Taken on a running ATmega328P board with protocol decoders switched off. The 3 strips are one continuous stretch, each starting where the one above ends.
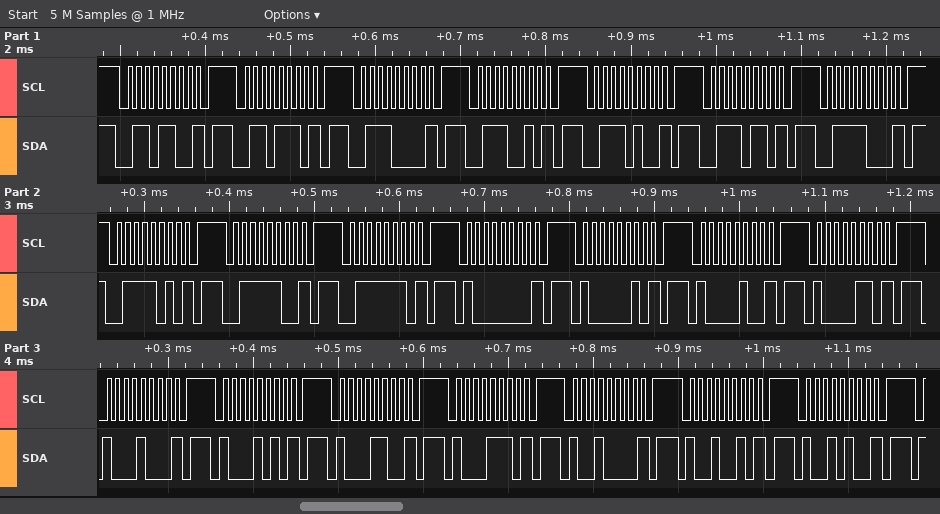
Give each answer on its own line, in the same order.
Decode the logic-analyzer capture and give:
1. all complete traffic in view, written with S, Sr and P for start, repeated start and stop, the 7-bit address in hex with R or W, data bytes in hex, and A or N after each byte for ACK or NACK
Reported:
S 36W N P S 37W N P S 38W N P S 39W N P S 3AW N P S 3BW N P S 3CW N P S 3DW N P S 3EW N P S 3FW N P S 40W N P S 41W N P S 42W N P S 43W N P S 44W N P S 45W N P S 46W N P S 47W N P S 48W N P S 49W N P S 4AW N P
